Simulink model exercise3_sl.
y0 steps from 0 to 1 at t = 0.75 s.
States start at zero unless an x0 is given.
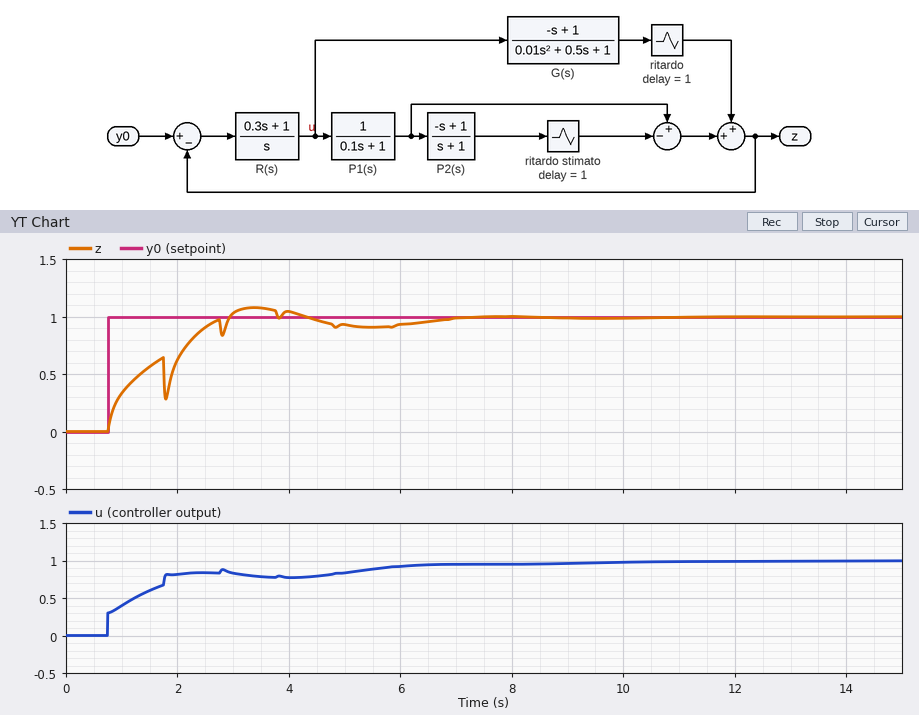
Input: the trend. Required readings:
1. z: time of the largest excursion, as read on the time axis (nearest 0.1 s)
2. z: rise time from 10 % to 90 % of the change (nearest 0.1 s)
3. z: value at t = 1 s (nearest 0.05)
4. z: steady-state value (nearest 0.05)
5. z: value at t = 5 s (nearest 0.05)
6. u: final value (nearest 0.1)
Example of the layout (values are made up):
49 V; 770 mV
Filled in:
3.4 s; 1.7 s; 0.35; 1.00; 0.95; 1.0
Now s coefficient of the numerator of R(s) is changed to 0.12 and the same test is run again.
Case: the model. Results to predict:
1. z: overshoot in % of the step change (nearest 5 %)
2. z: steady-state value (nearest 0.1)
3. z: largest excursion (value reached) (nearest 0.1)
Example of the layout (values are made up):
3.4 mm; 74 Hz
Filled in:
10 %; 1.0; 1.1
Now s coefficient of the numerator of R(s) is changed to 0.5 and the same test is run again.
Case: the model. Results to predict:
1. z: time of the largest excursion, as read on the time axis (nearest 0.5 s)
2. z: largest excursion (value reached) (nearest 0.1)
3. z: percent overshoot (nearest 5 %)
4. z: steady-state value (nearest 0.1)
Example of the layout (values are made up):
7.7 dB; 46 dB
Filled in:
4.0 s; 1.1; 10 %; 1.0
